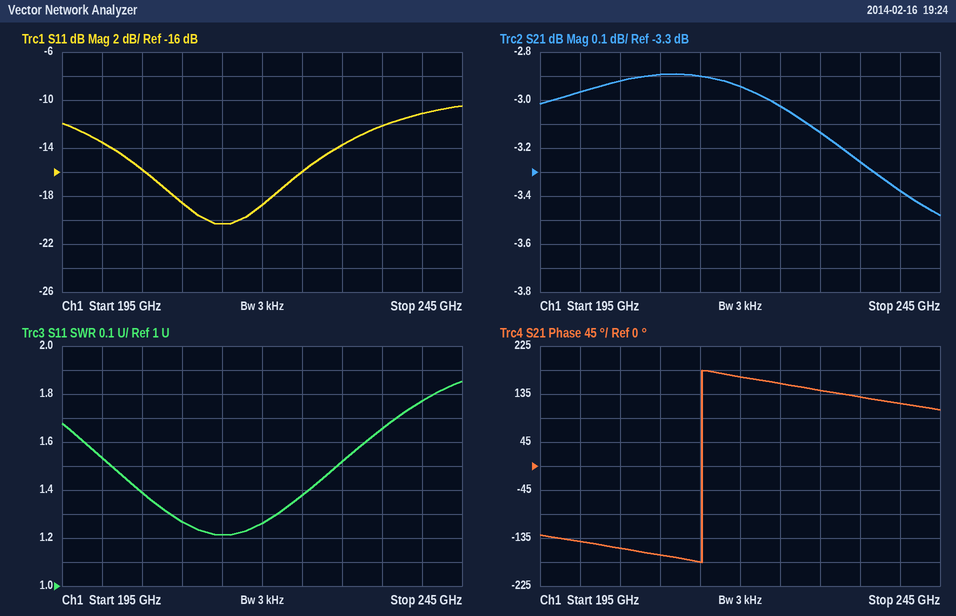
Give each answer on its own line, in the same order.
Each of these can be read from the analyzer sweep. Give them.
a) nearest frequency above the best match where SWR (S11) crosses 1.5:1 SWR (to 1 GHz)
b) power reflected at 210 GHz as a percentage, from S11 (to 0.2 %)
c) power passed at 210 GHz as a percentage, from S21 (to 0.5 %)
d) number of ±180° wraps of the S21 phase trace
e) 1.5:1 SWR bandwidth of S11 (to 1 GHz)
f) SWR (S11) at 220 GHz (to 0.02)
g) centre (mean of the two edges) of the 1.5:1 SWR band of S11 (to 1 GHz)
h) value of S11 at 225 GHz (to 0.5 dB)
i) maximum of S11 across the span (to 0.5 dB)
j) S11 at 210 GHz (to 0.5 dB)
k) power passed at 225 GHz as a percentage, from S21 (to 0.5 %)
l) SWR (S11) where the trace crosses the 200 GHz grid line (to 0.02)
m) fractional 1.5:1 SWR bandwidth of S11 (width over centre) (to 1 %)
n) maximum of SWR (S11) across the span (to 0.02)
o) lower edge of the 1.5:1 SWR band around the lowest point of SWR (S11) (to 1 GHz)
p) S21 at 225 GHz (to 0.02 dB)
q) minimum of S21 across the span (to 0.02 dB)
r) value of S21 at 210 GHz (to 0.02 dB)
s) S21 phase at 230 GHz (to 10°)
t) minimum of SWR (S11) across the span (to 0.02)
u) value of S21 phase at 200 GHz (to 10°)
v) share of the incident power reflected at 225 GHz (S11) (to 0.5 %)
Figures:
229 GHz
1.4 %
51.5 %
1
28 GHz
1.26
215 GHz
-16.0 dB
-10.5 dB
-18.5 dB
50.0 %
1.54
13 %
1.86
201 GHz
-3.02 dB
-3.48 dB
-2.90 dB
140°
1.22
-140°
2.5 %
